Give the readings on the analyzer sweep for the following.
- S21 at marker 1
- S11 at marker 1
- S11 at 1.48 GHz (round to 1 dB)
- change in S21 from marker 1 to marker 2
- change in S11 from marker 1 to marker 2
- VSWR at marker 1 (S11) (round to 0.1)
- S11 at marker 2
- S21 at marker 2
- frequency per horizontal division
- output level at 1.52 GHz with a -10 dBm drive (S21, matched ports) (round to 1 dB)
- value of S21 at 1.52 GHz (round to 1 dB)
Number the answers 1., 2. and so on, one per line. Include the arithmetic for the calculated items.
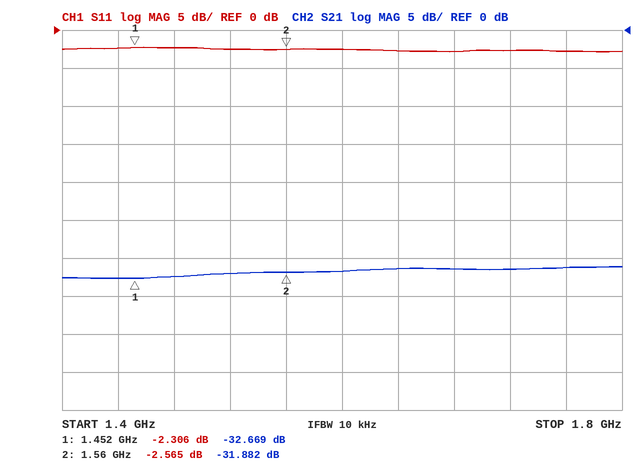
1. -32.669 dB
2. -2.306 dB
3. -2 dB
4. -31.882 − (-32.669) = 0.787 dB
5. -2.565 − (-2.306) = -0.259 dB
6. (1 + 0.7668)/(1 − 0.7668) ≈ 7.6
7. -2.565 dB
8. -31.882 dB
9. 40 MHz
10. -10 dBm + (-32 dB) = -42 dBm
11. -32 dB
